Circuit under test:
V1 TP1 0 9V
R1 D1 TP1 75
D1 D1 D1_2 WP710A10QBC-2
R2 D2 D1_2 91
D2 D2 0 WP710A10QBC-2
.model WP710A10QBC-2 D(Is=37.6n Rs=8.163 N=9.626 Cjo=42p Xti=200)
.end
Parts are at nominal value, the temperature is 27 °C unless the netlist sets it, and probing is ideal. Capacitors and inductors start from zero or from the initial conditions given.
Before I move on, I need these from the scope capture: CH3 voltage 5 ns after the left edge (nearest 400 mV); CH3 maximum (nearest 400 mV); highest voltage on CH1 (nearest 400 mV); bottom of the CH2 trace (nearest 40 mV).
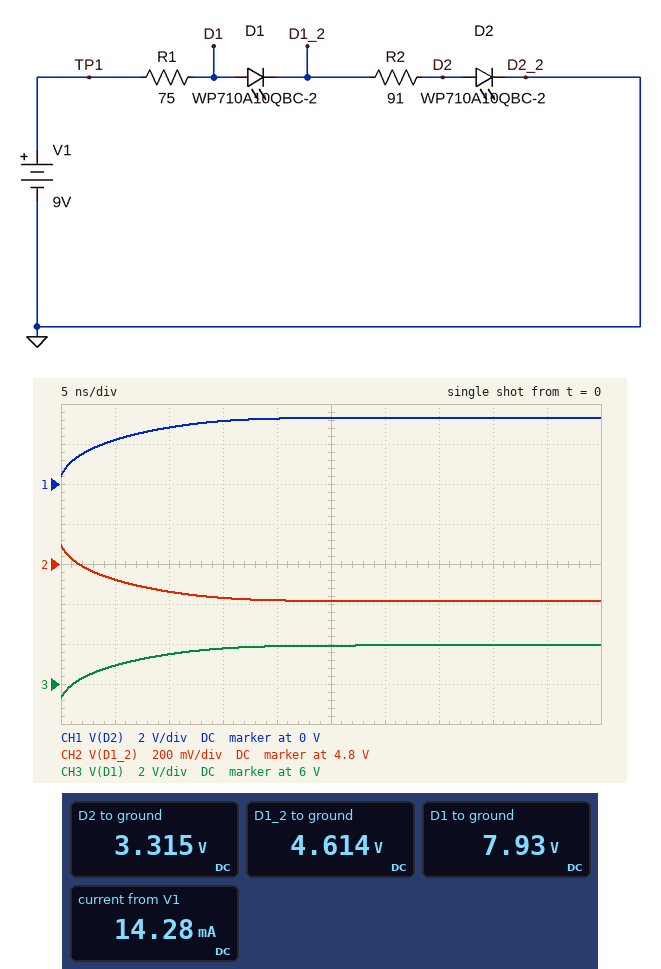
6.8 V
8.0 V
3.2 V
4.60 V
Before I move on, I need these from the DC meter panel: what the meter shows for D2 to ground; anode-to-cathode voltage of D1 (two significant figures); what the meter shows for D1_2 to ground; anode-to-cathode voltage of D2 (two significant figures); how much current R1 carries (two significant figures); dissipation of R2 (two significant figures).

3.315 V
3.3 V
4.614 V
3.3 V
14 mA
19 mW
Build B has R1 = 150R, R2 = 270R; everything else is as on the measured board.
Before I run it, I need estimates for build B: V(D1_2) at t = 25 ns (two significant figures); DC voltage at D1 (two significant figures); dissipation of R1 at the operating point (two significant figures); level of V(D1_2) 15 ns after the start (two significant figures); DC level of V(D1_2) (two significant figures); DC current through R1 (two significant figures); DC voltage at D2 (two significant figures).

5.0 V
8.0 V
7.0 mW
5.1 V
4.9 V
6.8 mA
3.1 V
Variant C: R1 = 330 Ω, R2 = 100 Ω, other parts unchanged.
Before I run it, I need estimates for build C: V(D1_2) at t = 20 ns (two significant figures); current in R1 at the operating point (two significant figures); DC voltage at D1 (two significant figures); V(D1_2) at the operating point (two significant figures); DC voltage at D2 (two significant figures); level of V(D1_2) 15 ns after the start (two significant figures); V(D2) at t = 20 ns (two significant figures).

3.4 V
6.7 mA
6.8 V
3.7 V
3.1 V
3.3 V
2.5 V
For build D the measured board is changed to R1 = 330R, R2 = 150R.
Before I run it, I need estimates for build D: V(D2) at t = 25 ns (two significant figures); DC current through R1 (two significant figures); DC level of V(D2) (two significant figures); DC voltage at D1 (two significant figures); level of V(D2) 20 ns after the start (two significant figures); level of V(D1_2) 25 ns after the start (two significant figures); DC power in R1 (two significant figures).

2.6 V
6.1 mA
3.0 V
7.0 V
2.4 V
3.8 V
12 mW
